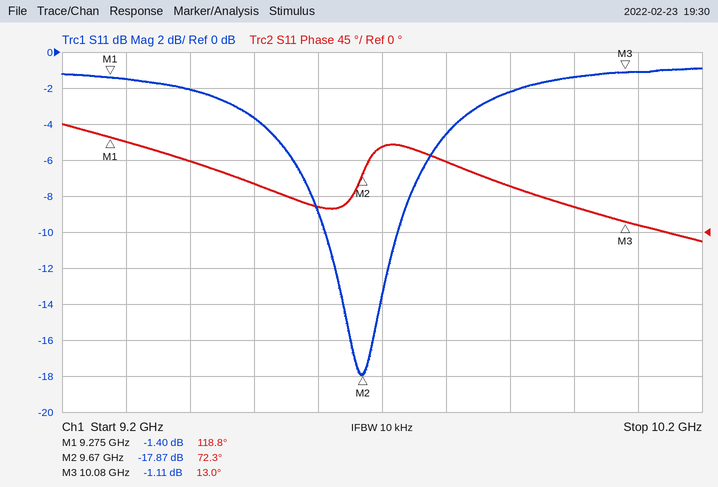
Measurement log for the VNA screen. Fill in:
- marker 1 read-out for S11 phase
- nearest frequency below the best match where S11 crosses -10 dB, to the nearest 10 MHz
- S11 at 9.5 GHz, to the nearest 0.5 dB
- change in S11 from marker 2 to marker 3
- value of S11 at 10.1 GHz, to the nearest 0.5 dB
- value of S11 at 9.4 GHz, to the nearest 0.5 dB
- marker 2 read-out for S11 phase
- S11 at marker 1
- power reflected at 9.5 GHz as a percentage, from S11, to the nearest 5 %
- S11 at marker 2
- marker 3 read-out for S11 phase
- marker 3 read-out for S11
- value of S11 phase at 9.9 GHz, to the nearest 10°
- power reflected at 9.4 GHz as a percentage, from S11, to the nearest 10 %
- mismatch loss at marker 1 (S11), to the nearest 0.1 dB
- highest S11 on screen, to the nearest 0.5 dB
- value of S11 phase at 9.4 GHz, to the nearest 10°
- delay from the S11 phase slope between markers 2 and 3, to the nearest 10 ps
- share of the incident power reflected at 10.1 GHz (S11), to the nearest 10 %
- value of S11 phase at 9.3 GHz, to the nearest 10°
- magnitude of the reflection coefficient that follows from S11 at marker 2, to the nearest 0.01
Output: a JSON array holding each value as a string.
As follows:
["118.8°", "9.61 GHz", "-3.5 dB", "16.76 dB", "-1.0 dB", "-2.0 dB", "72.3°", "-1.40 dB", "45 %", "-17.87 dB", "13.0°", "-1.11 dB", "60°", "60 %", "5.6 dB", "-1.0 dB", "90°", "400 ps", "80 %", "110°", "0.13"]
